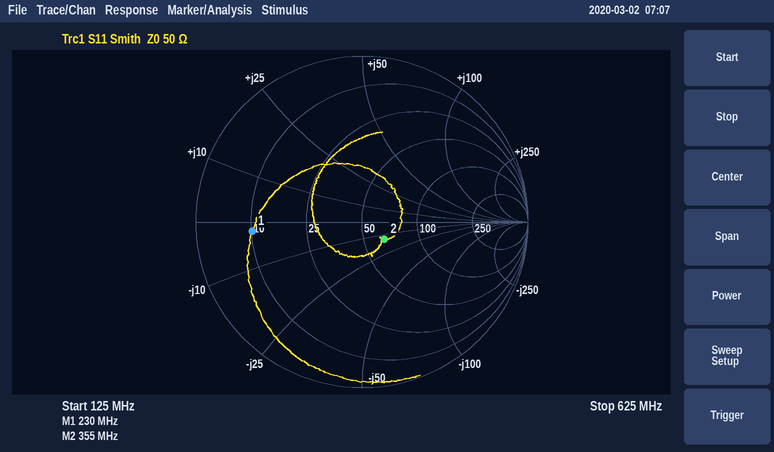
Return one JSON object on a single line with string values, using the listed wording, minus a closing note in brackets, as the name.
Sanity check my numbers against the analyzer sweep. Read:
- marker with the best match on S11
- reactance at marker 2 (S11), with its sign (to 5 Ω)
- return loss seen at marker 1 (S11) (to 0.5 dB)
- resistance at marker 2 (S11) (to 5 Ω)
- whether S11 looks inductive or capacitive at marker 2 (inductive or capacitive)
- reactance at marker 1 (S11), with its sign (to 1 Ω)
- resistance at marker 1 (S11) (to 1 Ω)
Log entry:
{"marker with the best match on S11": "marker 2", "reactance at marker 2 (S11), with its sign": "-15 Ω", "return loss seen at marker 1 (S11)": "3.5 dB", "resistance at marker 2 (S11)": "65 Ω", "whether S11 looks inductive or capacitive at marker 2": "capacitive", "reactance at marker 1 (S11), with its sign": "-2 Ω", "resistance at marker 1 (S11)": "10 Ω"}
